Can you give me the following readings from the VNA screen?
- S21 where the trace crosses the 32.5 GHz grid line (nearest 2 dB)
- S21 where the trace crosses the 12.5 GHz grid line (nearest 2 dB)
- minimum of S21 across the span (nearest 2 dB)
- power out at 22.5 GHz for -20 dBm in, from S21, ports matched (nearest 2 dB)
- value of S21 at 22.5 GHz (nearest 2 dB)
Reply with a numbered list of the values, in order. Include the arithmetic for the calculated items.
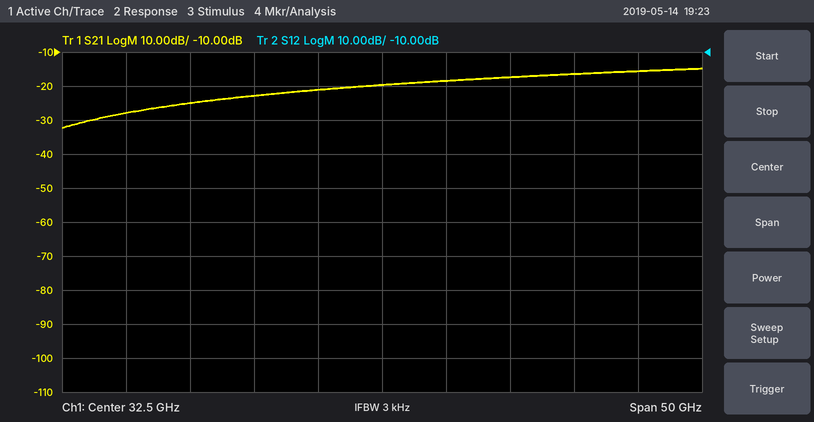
1. -20 dB
2. -28 dB
3. -32 dB
4. -20 dBm + (-22 dB) = -42 dBm
5. -22 dB
